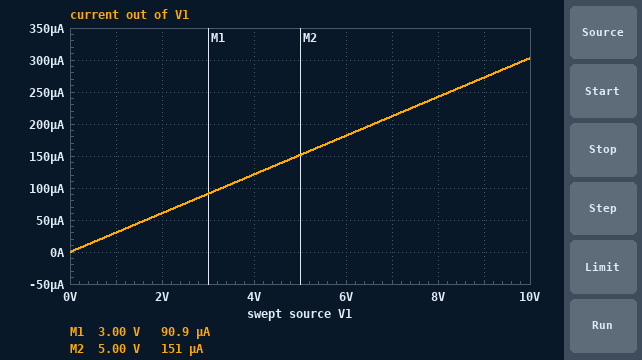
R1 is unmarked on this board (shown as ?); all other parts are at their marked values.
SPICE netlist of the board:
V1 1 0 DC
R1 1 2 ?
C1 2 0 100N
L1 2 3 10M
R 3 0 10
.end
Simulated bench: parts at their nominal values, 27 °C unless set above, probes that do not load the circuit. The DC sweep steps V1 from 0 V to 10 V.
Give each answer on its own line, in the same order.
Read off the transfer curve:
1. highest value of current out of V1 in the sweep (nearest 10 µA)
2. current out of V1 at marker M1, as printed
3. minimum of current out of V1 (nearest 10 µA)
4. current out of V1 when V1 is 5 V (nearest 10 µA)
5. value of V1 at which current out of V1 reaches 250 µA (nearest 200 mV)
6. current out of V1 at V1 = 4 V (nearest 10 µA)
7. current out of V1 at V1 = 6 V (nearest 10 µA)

300 µA
90.9 µA
0 A
150 µA
8.2 V
120 µA
180 µA
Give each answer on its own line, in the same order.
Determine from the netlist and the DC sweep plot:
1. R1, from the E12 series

33 kΩ
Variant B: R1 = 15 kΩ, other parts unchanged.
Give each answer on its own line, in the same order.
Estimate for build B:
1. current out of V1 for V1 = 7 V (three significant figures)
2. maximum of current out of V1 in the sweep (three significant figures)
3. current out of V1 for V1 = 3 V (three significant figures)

466 µA
666 µA
200 µA
